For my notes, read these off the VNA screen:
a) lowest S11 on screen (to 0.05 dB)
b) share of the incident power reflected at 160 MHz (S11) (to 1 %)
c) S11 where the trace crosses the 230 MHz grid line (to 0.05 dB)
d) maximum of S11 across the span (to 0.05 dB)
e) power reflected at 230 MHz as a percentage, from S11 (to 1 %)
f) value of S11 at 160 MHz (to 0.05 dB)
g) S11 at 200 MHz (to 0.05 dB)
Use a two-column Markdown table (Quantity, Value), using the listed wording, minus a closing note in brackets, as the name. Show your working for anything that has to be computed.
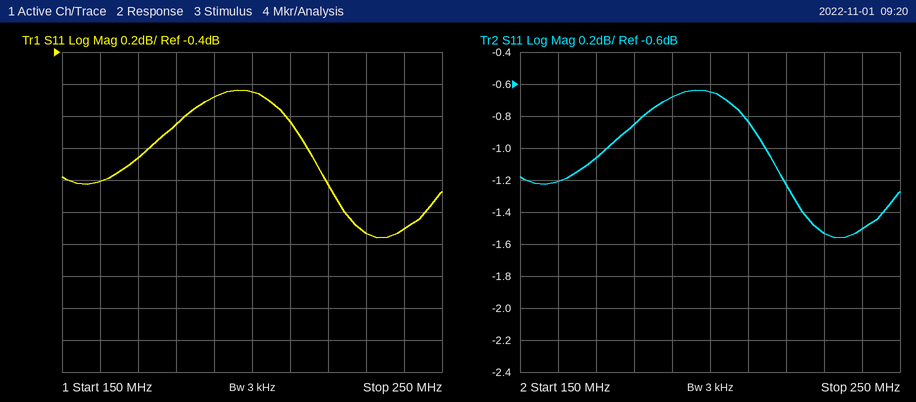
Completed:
| Quantity | Value |
|---|---|
| lowest S11 on screen | -1.55 dB |
| share of the incident power reflected at 160 MHz (S11) | 10^(-1.2/10) ≈ 76 % |
| S11 where the trace crosses the 230 MHz grid line | -1.55 dB |
| maximum of S11 across the span | -0.65 dB |
| power reflected at 230 MHz as a percentage, from S11 | 10^(-1.55/10) ≈ 70 % |
| value of S11 at 160 MHz | -1.20 dB |
| S11 at 200 MHz | -0.65 dB |
